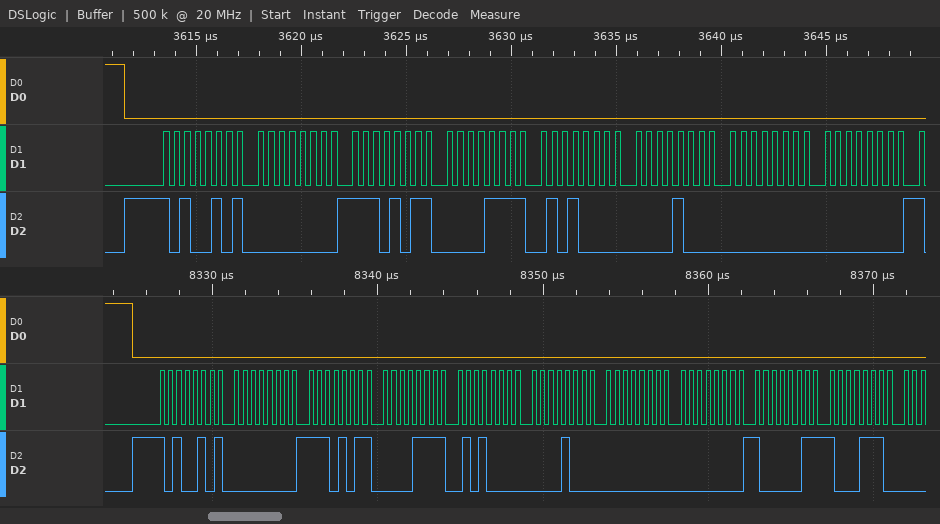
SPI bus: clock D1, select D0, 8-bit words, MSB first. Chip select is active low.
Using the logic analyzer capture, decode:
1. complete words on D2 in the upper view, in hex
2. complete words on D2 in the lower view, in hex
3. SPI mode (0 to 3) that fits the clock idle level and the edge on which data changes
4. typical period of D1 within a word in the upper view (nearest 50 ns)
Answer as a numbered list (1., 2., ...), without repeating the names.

1. A5, 00, EB, 0F, 50, 08, 00, 00
2. A5, 00, EB, 0F, 50, 08, 00, 00, 83, 8E
3. 0
4. 500 ns
